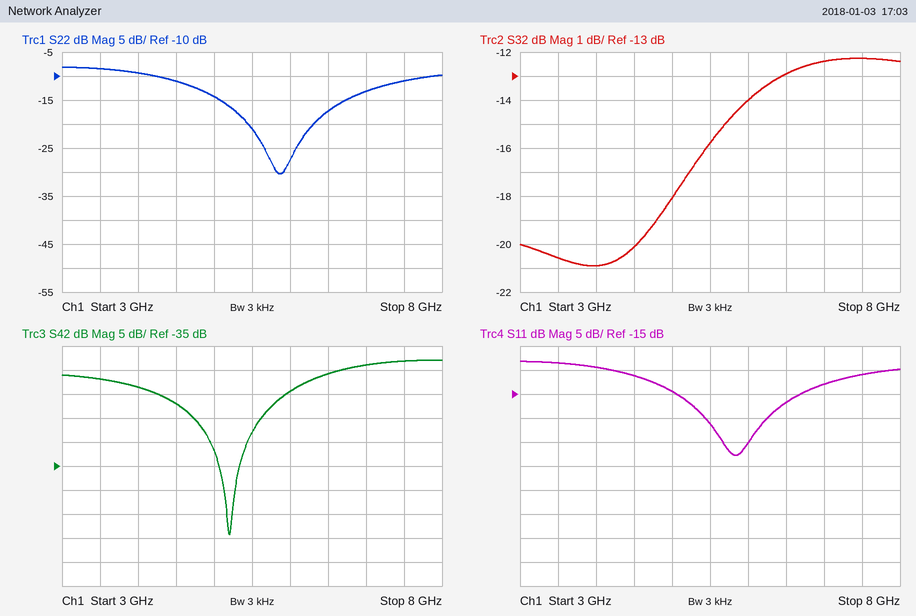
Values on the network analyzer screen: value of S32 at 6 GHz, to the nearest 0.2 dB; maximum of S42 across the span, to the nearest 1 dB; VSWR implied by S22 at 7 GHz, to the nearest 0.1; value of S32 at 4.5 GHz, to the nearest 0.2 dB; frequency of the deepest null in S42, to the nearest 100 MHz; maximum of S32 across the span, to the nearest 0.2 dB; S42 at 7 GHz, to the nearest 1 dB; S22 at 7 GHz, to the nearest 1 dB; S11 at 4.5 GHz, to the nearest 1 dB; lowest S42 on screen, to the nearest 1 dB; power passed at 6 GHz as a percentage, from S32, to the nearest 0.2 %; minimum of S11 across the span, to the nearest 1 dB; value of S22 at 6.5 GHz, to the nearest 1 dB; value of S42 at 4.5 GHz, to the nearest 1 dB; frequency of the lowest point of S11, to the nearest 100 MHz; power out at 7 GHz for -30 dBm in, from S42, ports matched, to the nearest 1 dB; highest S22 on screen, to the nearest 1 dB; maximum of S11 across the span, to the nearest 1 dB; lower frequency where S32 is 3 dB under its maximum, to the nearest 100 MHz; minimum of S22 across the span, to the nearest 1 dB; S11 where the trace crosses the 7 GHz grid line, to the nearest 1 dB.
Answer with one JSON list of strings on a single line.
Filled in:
["-14.0 dB", "-13 dB", "1.6", "-20.2 dB", "5.2 GHz", "-12.2 dB", "-14 dB", "-13 dB", "-11 dB", "-49 dB", "4.0 %", "-28 dB", "-17 dB", "-22 dB", "5.8 GHz", "-44 dBm", "-8 dB", "-8 dB", "5.6 GHz", "-30 dB", "-13 dB"]
